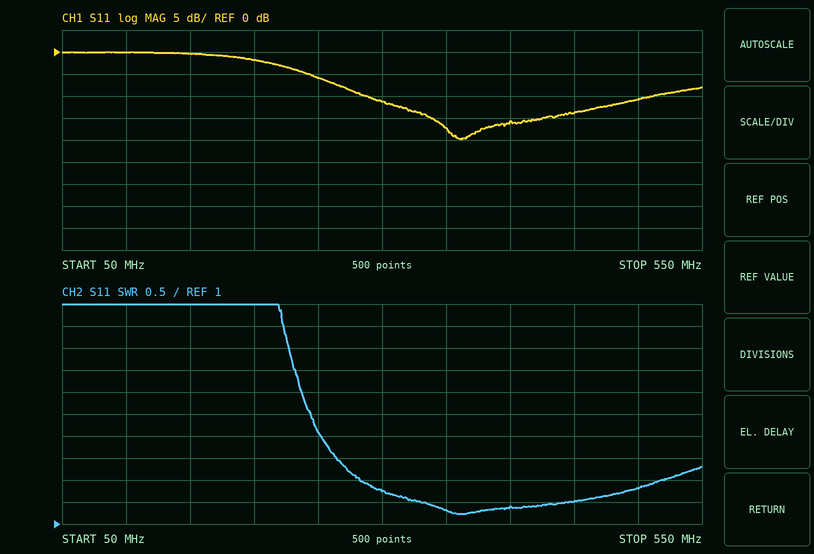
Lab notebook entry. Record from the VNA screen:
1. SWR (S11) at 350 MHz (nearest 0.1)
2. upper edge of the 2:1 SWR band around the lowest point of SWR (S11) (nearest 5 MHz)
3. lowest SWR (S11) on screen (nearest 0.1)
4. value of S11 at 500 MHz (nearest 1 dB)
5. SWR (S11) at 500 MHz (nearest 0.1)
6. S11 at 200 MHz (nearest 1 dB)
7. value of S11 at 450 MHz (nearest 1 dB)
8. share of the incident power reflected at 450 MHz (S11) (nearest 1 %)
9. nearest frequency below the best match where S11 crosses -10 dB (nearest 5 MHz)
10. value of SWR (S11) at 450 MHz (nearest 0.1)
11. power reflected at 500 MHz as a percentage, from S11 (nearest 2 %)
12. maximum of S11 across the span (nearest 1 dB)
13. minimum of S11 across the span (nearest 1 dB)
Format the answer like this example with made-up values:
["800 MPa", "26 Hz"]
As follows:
["1.3", "520 MHz", "1.2", "-11 dB", "1.8", "-2 dB", "-14 dB", "4 %", "290 MHz", "1.5", "8 %", "0 dB", "-20 dB"]
